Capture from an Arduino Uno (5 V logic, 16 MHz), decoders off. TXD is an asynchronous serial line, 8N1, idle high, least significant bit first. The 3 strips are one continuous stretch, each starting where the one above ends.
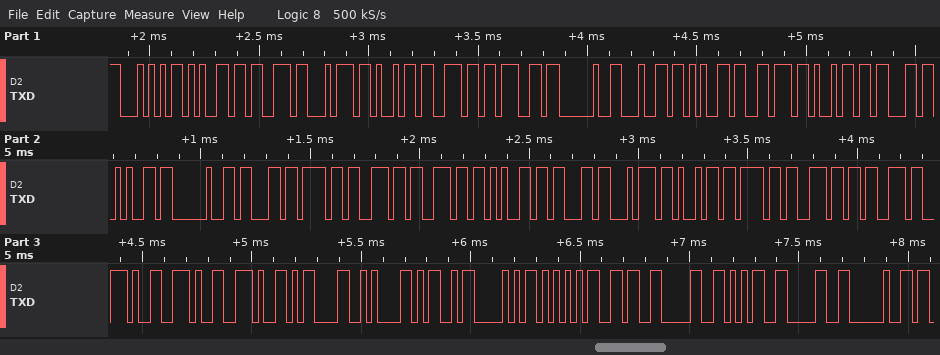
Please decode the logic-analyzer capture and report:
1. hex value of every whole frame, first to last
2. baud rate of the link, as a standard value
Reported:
0x54 0x65 0x73 0x74 0x69 0x6E 0x67 0x20 0x64 0x65 0x76 0x69 0x63 0x65 0x20 0x63 0x6F 0x6E 0x6E 0x65 0x63 0x74 0x69 0x6F 0x6E 0x73 0x2E 0x2E 0x2E 0x0D 0x0A 0x4D 0x50 0x55 0x36 0x30 0x35 0x30 0x20
38400 baud
